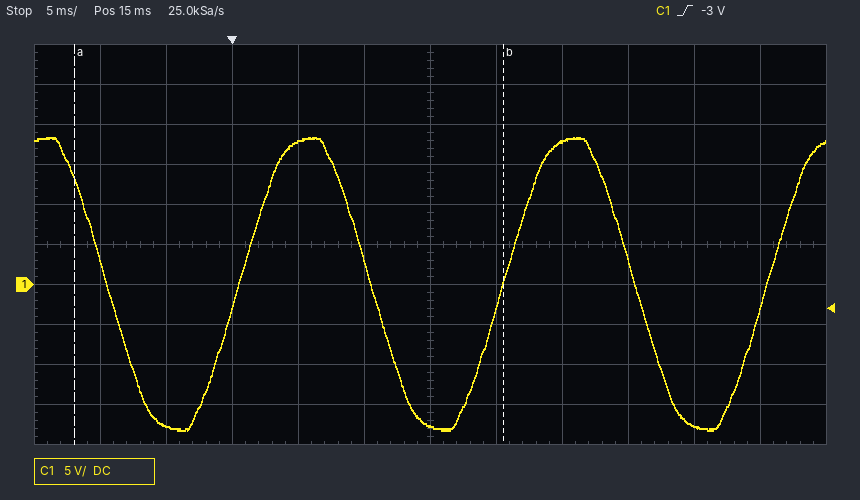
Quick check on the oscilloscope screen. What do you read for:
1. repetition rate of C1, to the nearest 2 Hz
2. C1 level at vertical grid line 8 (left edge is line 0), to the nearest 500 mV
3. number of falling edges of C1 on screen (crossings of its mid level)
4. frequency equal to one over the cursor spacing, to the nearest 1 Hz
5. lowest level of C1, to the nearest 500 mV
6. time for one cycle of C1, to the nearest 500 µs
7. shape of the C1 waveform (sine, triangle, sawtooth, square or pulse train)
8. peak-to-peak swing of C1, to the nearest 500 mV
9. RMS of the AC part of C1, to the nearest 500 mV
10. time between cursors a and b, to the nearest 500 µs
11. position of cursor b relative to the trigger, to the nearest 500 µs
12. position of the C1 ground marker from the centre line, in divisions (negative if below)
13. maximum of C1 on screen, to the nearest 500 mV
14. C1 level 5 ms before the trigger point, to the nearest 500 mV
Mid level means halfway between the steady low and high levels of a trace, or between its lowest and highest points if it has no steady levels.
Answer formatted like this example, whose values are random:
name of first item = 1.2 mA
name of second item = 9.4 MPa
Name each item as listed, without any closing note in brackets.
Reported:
repetition rate of C1, to the nearest 2 Hz = 50 Hz
C1 level at vertical grid line 8 (left edge is line 0), to the nearest 500 mV = 18.0 V
number of falling edges of C1 on screen = 3
frequency equal to one over the cursor spacing, to the nearest 1 Hz = 31 Hz
lowest level of C1, to the nearest 500 mV = -18.0 V
time for one cycle of C1, to the nearest 500 µs = 20.0 ms
shape of the C1 waveform = sine
peak-to-peak swing of C1, to the nearest 500 mV = 36.5 V
RMS of the AC part of C1, to the nearest 500 mV = 13.0 V
time between cursors a and b, to the nearest 500 µs = 32.5 ms
position of cursor b relative to the trigger, to the nearest 500 µs = +20.5 ms
position of the C1 ground marker from the centre line, in divisions = -1.0 div
maximum of C1 on screen, to the nearest 500 mV = 18.5 V
C1 level 5 ms before the trigger point, to the nearest 500 mV = -17.5 V
